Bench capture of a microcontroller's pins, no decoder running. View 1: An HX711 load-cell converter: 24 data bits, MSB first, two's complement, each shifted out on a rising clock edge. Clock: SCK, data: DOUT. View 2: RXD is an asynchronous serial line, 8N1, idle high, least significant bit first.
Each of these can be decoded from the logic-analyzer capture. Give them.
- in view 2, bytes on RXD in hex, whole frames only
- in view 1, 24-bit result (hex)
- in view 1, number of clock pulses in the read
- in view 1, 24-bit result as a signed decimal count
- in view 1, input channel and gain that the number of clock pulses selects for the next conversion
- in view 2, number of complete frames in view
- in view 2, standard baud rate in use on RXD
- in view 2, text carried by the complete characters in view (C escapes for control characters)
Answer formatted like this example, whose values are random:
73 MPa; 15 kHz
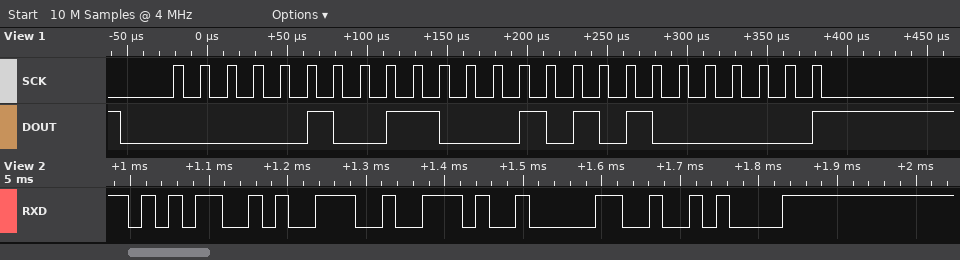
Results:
0x35 0x39 0x2E 0x30 0x0A; 0x04C540; 25; 312640; channel A, gain 128; 5; 57600 baud; "59.0\n"
